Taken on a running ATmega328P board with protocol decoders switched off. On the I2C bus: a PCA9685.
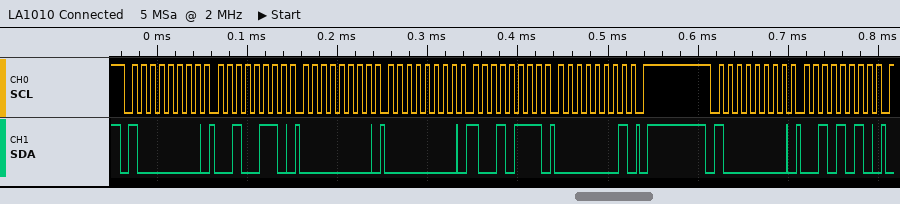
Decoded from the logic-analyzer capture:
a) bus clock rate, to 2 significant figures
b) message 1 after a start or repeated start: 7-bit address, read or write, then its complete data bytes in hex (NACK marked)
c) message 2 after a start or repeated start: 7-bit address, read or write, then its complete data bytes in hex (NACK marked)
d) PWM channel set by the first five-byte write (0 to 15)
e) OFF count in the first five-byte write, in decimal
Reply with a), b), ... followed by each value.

a) 100 kHz
b) 0x40 write: 26 00 00 97 01
c) 0x40 write: 2A
d) 8
e) 407
